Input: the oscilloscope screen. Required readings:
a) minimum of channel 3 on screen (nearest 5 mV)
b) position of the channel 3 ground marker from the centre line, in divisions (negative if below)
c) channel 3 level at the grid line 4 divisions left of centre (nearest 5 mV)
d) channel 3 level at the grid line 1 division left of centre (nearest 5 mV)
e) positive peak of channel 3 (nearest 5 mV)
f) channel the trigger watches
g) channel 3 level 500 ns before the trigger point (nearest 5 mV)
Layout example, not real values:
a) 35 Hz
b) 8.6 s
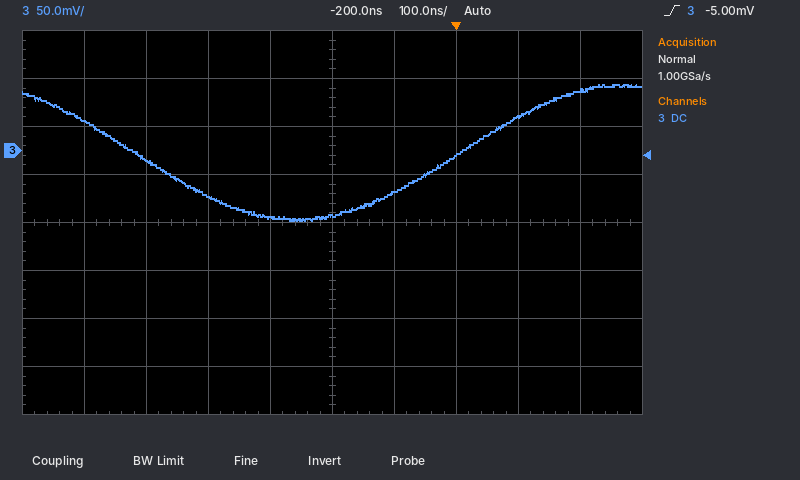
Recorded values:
a) -75 mV
b) +1.5 div
c) 30 mV
d) -70 mV
e) 70 mV
f) channel 3
g) -10 mV
